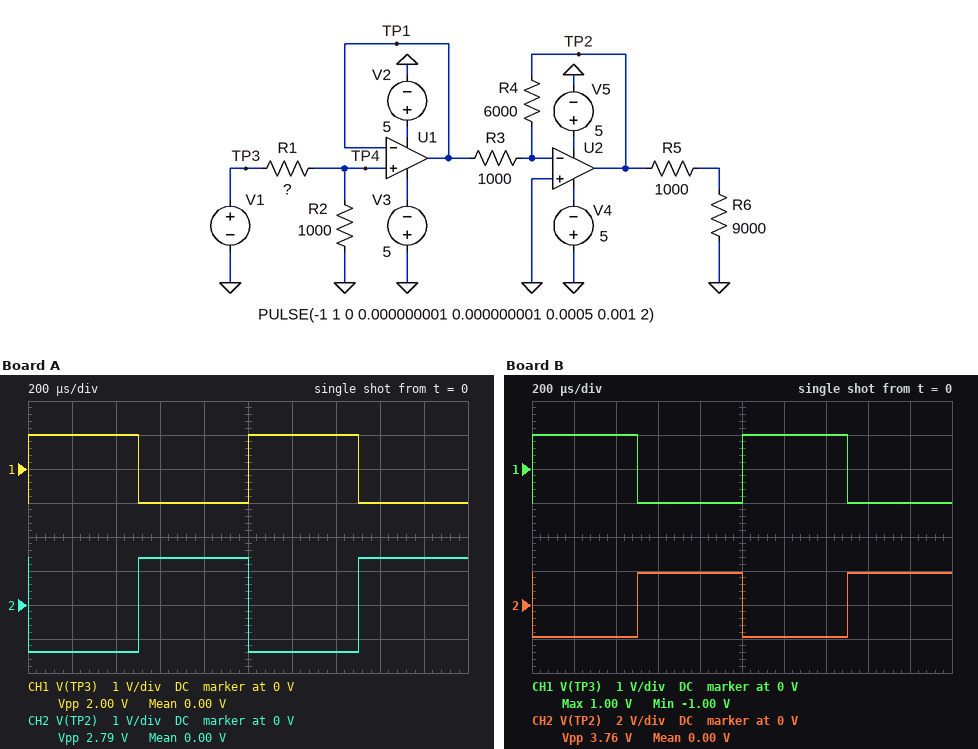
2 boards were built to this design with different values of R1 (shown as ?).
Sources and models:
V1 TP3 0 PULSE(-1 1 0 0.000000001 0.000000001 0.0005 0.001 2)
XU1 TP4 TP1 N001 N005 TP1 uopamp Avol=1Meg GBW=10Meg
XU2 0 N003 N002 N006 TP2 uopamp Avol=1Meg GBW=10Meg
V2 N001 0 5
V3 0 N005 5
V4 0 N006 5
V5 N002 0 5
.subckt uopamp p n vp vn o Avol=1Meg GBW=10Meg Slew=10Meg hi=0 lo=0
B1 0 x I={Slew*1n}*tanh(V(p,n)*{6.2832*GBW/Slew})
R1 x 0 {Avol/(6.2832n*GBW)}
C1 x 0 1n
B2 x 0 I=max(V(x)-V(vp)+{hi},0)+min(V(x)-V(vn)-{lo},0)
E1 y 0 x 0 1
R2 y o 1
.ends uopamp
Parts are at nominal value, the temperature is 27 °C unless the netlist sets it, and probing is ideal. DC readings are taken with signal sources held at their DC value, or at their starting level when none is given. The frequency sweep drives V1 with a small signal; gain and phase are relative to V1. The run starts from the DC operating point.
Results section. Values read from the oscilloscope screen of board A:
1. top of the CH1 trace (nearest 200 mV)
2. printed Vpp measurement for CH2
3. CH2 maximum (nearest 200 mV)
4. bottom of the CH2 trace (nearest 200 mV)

1.0 V
2.79 V
1.4 V
-1.4 V
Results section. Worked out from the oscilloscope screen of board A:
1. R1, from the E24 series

3.3 kΩ
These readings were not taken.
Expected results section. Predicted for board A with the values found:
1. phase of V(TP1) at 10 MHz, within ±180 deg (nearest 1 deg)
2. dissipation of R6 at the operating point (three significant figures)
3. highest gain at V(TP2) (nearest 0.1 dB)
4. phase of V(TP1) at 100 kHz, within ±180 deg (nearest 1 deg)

-45 deg
175 µW
2.9 dB
-1 deg
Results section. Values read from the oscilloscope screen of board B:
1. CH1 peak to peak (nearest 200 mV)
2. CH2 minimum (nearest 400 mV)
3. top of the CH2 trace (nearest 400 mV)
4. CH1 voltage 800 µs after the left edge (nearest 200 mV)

2.0 V
-2.0 V
2.0 V
-1.0 V
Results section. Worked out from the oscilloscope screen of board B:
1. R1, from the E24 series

2.2 kΩ
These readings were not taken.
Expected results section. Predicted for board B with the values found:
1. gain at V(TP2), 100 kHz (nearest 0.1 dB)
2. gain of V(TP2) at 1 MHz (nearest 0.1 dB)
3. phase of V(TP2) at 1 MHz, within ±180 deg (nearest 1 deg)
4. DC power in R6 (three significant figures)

5.4 dB
3.7 dB
139 deg
316 µW
